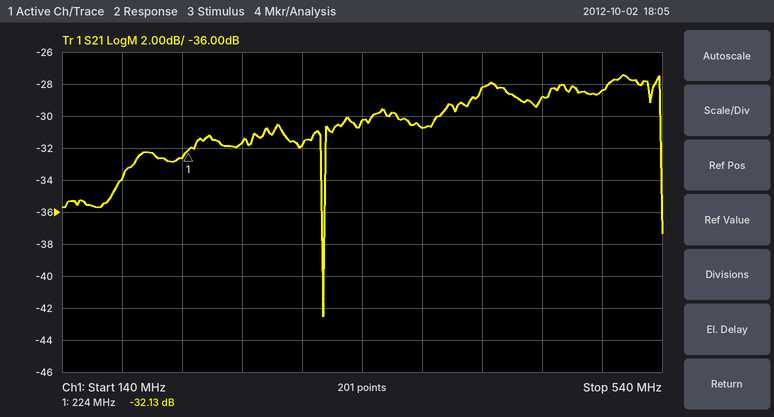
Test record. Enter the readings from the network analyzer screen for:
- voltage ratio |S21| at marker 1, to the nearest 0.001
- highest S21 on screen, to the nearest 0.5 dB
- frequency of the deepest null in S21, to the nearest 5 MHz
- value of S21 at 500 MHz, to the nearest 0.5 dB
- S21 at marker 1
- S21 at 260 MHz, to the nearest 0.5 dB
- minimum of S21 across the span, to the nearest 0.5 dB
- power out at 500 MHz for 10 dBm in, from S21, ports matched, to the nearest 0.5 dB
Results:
0.025
-27.5 dB
315 MHz
-28.5 dB
-32.13 dB
-31.5 dB
-42.5 dB
-18.5 dBm
